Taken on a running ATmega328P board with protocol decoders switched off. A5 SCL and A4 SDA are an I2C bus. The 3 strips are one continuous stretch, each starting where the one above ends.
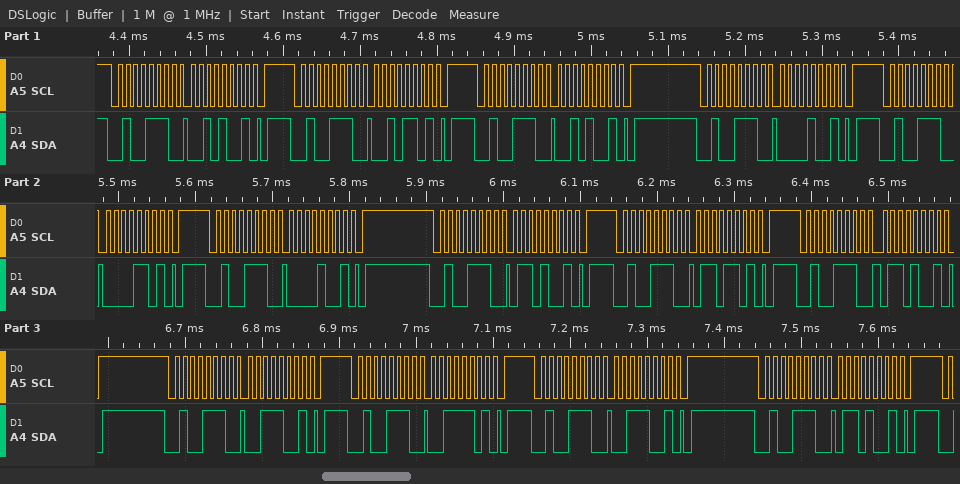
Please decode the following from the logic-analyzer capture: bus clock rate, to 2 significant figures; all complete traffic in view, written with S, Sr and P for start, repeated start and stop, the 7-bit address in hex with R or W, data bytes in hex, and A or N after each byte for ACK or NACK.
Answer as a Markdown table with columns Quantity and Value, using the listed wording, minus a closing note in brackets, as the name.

| Quantity | Value |
|---|---|
| bus clock rate, to 2 significant figures | 100 kHz |
| all complete traffic in view, written with S, Sr and P for start, repeated start and stop, the 7-bit address in hex with R or W, data bytes in hex, and A or N after each byte for ACK or NACK | S 27W A 29 A P S 27W A 2D A P S 27W A 29 A P S 27W A 09 A P S 27W A 0D A P S 27W A 09 A P S 27W A 69 A P S 27W A 6D A P S 27W A 69 A P S 27W A 39 A P S 27W A 3D A P S 27W A 39 A P S 27W A 69 A P |
